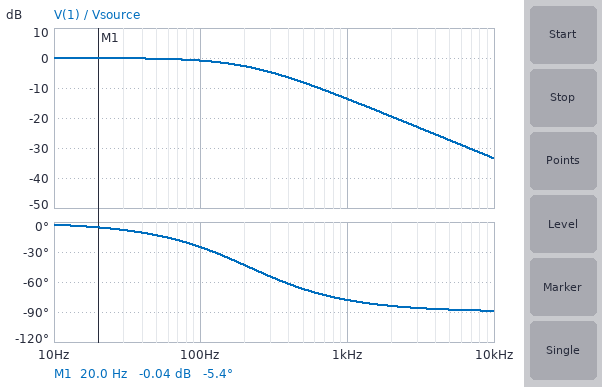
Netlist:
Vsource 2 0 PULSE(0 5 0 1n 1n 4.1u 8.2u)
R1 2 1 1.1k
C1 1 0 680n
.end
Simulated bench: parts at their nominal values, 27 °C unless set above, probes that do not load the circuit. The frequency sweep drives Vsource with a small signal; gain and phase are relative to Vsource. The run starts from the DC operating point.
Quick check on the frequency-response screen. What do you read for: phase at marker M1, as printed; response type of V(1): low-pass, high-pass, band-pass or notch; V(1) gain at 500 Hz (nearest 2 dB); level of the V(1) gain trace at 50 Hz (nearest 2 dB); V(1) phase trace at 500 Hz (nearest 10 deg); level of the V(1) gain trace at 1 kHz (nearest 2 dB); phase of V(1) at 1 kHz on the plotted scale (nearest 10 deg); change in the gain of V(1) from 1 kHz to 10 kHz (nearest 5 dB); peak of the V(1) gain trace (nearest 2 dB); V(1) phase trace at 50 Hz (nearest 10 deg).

-5.4 deg
low-pass
-8 dB
0 dB
-70 deg
-14 dB
-80 deg
-20 dB
0 dB
-10 deg
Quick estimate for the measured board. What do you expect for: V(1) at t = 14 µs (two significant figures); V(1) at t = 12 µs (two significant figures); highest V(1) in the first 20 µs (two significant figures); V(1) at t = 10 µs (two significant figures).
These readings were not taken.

54 mV
52 mV
78 mV
39 mV
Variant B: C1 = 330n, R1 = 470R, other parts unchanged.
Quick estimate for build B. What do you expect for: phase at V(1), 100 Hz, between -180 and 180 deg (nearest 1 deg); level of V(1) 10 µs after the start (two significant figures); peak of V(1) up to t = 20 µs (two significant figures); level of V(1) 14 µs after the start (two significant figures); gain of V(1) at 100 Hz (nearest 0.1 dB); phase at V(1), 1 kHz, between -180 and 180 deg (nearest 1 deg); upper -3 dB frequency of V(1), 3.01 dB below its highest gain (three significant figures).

-6 deg
180 mV
360 mV
250 mV
0 dB
-44 deg
1.03 kHz
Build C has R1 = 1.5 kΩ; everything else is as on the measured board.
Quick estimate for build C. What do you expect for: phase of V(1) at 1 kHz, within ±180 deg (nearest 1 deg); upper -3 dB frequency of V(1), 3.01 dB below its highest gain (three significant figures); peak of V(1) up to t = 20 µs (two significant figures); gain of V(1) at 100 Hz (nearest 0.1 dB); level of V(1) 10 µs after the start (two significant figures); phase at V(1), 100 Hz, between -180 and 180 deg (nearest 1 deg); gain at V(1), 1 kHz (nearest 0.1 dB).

-81 deg
156 Hz
57 mV
-1.5 dB
29 mV
-33 deg
-16.2 dB
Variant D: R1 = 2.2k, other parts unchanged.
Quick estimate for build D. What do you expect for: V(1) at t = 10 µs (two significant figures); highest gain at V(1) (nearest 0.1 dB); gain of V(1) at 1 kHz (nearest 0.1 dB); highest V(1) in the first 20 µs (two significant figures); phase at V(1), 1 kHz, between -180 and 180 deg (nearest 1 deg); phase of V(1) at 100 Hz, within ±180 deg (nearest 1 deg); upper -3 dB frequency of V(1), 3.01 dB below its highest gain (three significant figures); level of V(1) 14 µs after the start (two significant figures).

20 mV
0 dB
-19.5 dB
39 mV
-84 deg
-43 deg
106 Hz
27 mV
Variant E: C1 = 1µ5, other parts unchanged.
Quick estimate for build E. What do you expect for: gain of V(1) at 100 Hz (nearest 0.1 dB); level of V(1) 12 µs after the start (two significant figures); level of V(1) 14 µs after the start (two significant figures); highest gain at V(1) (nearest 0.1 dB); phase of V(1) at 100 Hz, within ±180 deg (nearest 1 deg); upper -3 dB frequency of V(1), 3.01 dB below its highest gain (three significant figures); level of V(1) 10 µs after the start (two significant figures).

-3.2 dB
24 mV
25 mV
0 dB
-46 deg
96.5 Hz
18 mV
